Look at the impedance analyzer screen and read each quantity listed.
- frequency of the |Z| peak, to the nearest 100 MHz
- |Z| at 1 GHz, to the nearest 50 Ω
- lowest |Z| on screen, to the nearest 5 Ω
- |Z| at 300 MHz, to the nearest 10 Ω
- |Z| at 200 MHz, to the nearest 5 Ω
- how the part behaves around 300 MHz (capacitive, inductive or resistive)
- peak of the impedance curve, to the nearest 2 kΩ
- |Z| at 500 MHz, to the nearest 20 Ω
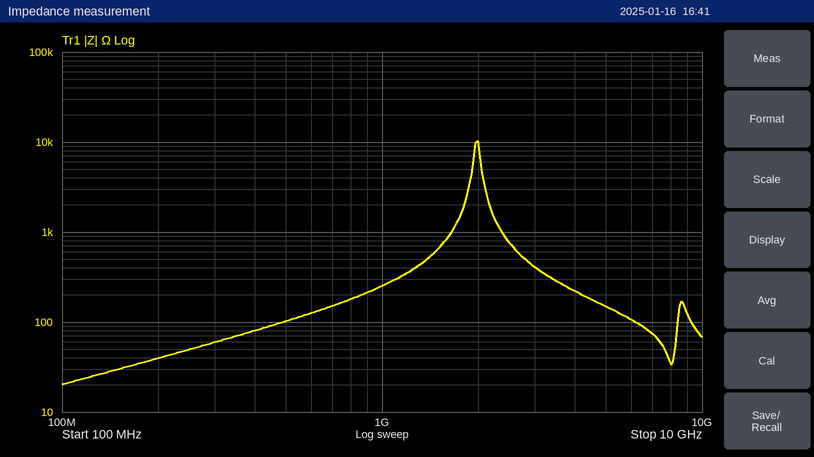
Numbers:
2.0 GHz
250 Ω
20 Ω
60 Ω
40 Ω
inductive
10 kΩ
100 Ω
